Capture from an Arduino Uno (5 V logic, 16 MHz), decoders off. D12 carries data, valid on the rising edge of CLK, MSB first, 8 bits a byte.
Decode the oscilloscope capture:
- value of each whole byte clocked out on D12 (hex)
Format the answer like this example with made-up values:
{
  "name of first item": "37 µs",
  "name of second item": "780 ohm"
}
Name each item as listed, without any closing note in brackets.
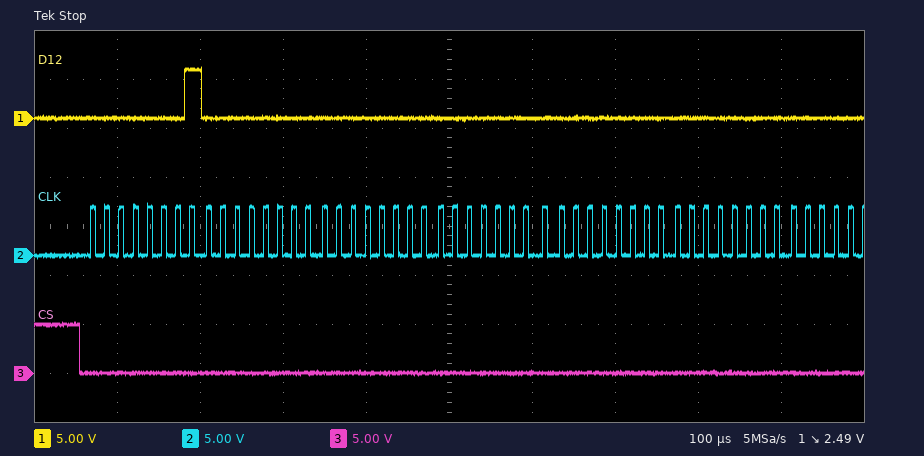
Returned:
{
  "value of each whole byte clocked out on D12": "01 00 00 00 00 00"
}
